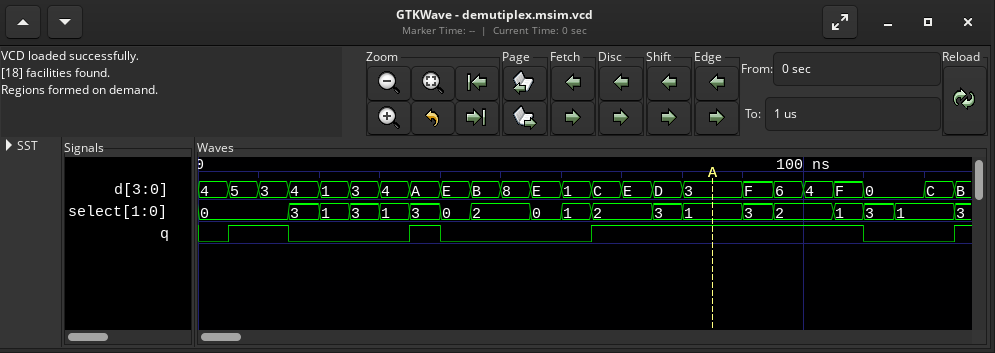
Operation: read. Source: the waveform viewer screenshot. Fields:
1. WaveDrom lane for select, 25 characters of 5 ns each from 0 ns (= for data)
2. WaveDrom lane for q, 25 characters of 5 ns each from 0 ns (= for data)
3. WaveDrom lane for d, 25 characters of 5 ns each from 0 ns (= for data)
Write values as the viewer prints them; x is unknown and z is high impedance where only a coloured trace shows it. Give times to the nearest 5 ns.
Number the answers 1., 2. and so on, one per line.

1. {name: 'select', wave: '=..=======.===.==.==.===.', data: '0 3 1 3 1 3 0 2 0 1 2 3 1 3 2 1 3 1'}
2. {name: 'q', wave: '01.0...10....1........0..'}
3. {name: 'd', wave: '=================.=====.=', data: '4 5 3 4 1 3 4 A E B 8 E 1 C E D 3 F 6 4 F 0 C'}
